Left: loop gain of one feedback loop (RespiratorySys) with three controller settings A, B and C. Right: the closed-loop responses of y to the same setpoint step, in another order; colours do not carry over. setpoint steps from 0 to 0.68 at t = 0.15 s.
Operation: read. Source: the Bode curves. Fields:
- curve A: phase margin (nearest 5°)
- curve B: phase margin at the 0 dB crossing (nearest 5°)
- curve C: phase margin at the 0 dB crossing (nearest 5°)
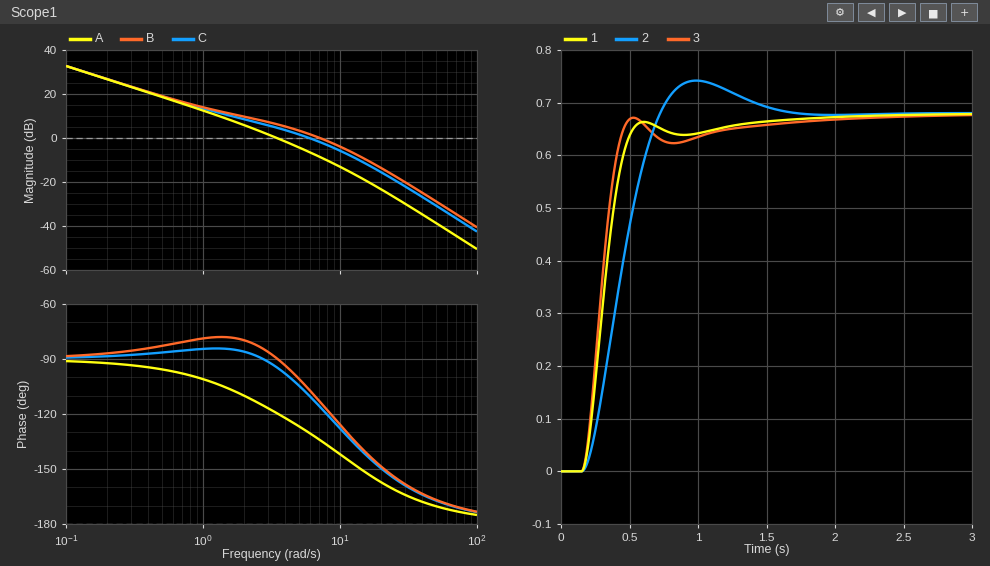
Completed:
60°
65°
70°
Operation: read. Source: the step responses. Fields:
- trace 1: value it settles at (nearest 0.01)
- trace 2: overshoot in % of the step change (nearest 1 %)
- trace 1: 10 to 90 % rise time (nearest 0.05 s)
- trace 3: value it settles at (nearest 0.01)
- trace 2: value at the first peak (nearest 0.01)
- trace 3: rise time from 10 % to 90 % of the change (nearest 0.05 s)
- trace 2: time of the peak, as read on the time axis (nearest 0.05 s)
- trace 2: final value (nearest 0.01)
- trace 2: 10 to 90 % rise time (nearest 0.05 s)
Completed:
0.68
9 %
0.25 s
0.68
0.74
0.20 s
1.00 s
0.68
0.40 s
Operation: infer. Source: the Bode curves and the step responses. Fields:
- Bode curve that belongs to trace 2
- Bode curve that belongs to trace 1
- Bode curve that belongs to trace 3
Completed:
A
C
B
